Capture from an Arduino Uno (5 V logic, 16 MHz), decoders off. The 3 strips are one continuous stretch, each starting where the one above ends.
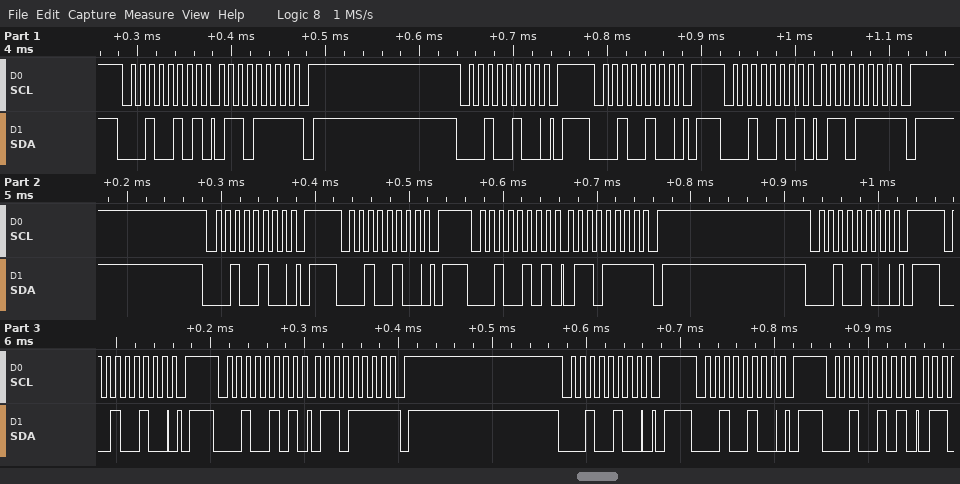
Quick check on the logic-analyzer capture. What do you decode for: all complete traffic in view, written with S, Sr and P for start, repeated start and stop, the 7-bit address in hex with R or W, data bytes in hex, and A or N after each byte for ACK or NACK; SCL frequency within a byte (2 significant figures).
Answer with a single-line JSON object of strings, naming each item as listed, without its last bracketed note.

{"all complete traffic in view, written with S, Sr and P for start, repeated start and stop, the 7-bit address in hex with R or W, data bytes in hex, and A or N after each byte for ACK or NACK": "S 12R A 6F N P S 12W A P S 12W A P S 12R A 6F N P S 12W A P S 12W A P S 12R A 6F N P S 12W A P S 12W A P S 12R A 6F N P S 12W A P S 12W A P S 12R A", "SCL frequency within a byte": "100 kHz"}
